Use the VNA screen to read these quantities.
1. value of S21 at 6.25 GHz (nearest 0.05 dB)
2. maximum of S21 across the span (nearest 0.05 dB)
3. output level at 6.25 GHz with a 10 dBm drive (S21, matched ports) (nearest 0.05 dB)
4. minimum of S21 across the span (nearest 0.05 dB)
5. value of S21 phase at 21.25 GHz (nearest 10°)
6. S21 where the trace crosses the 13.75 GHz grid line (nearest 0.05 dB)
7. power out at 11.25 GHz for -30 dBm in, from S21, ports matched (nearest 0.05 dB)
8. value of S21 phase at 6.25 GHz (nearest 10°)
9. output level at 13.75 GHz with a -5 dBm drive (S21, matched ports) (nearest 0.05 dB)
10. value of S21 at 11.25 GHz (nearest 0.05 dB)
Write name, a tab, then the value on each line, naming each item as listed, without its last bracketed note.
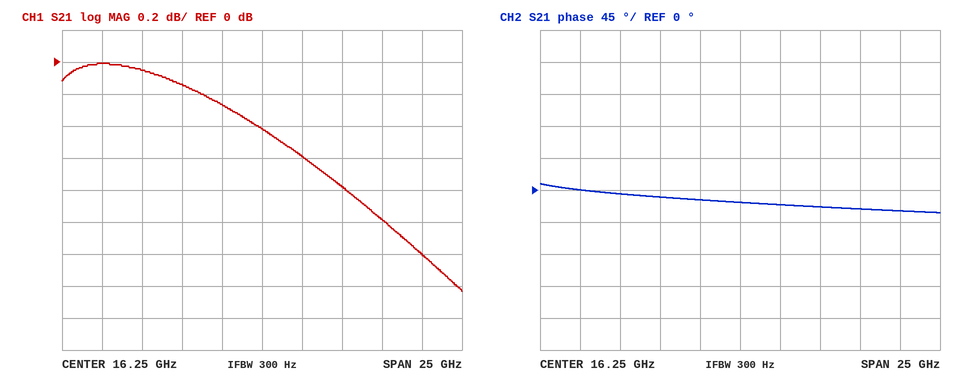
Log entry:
value of S21 at 6.25 GHz	0.00 dB
maximum of S21 across the span	0.00 dB
output level at 6.25 GHz with a 10 dBm drive (S21, matched ports)	10.00 dBm
minimum of S21 across the span	-1.45 dB
value of S21 phase at 21.25 GHz	-20°
S21 where the trace crosses the 13.75 GHz grid line	-0.25 dB
power out at 11.25 GHz for -30 dBm in, from S21, ports matched	-30.15 dBm
value of S21 phase at 6.25 GHz	0°
output level at 13.75 GHz with a -5 dBm drive (S21, matched ports)	-5.25 dBm
value of S21 at 11.25 GHz	-0.15 dB
